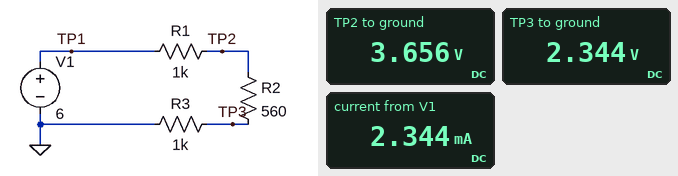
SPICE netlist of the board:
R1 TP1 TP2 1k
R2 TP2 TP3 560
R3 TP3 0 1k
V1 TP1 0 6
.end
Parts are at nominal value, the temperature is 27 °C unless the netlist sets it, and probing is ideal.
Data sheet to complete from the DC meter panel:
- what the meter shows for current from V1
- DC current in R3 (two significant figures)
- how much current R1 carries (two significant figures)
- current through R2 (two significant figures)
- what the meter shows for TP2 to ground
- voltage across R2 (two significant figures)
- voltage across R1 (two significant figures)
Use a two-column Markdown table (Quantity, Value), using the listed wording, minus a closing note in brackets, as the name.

| Quantity | Value |
|---|---|
| what the meter shows for current from V1 | 2.344 mA |
| DC current in R3 | 2.3 mA |
| how much current R1 carries | 2.3 mA |
| current through R2 | 2.3 mA |
| what the meter shows for TP2 to ground | 3.656 V |
| voltage across R2 | 1.3 V |
| voltage across R1 | 2.3 V |
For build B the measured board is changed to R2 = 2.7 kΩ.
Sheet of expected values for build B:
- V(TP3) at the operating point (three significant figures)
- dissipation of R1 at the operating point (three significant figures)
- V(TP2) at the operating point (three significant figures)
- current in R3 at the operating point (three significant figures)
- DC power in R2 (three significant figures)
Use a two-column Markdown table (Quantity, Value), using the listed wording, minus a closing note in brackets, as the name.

| Quantity | Value |
|---|---|
| V(TP3) at the operating point | 1.28 V |
| dissipation of R1 at the operating point | 1.63 mW |
| V(TP2) at the operating point | 4.72 V |
| current in R3 at the operating point | 1.28 mA |
| DC power in R2 | 4.40 mW |
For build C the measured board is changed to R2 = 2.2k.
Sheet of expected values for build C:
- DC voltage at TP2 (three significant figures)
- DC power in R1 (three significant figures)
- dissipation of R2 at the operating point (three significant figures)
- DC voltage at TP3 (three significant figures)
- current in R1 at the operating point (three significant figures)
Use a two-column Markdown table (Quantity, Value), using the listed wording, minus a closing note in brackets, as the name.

| Quantity | Value |
|---|---|
| DC voltage at TP2 | 4.57 V |
| DC power in R1 | 2.04 mW |
| dissipation of R2 at the operating point | 4.49 mW |
| DC voltage at TP3 | 1.43 V |
| current in R1 at the operating point | 1.43 mA |
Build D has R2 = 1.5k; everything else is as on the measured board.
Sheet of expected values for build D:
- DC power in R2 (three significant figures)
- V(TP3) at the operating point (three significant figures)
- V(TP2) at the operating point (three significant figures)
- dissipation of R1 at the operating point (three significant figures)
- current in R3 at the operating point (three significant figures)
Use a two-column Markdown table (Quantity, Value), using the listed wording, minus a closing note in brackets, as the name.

| Quantity | Value |
|---|---|
| DC power in R2 | 4.41 mW |
| V(TP3) at the operating point | 1.71 V |
| V(TP2) at the operating point | 4.29 V |
| dissipation of R1 at the operating point | 2.94 mW |
| current in R3 at the operating point | 1.71 mA |
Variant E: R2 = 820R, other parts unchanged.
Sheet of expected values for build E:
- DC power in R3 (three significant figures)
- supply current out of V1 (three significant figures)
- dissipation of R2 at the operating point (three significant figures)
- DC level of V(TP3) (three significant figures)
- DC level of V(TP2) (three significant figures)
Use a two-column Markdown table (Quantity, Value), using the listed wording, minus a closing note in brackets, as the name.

| Quantity | Value |
|---|---|
| DC power in R3 | 4.53 mW |
| supply current out of V1 | 2.13 mA |
| dissipation of R2 at the operating point | 3.71 mW |
| DC level of V(TP3) | 2.13 V |
| DC level of V(TP2) | 3.87 V |
